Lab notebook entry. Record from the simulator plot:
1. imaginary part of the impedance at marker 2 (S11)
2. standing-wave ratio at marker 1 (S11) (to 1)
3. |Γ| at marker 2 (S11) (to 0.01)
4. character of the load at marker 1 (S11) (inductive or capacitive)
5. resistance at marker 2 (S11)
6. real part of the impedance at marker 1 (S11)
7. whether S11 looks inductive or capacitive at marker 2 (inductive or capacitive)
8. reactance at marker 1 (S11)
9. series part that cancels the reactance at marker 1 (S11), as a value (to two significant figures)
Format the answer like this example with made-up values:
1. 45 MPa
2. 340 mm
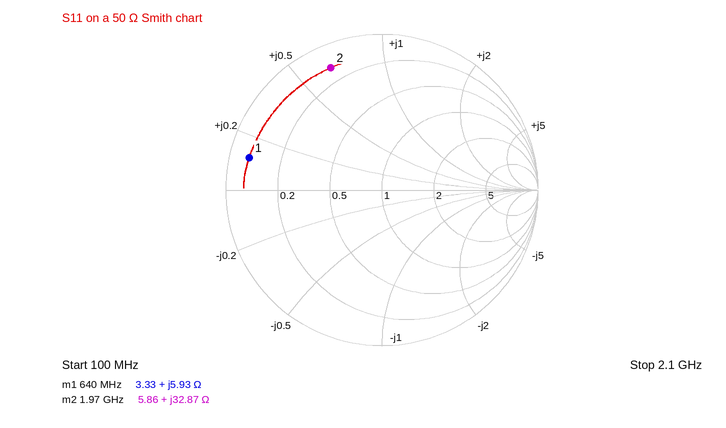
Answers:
1. +32.87 Ω
2. 15
3. 0.85
4. inductive
5. 5.86 Ω
6. 3.33 Ω
7. inductive
8. +5.93 Ω
9. 42 pF
